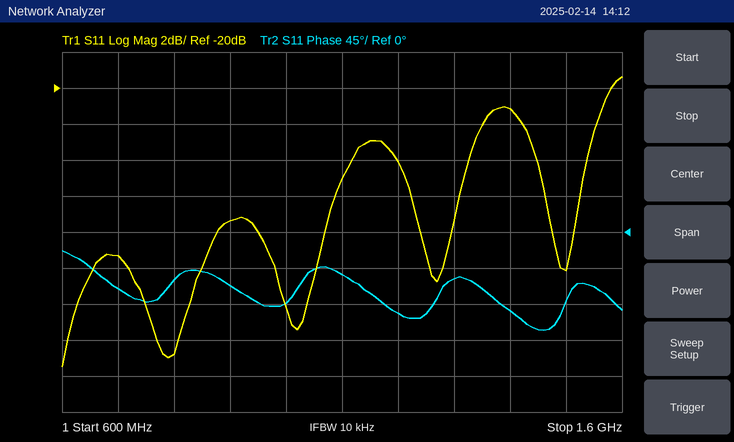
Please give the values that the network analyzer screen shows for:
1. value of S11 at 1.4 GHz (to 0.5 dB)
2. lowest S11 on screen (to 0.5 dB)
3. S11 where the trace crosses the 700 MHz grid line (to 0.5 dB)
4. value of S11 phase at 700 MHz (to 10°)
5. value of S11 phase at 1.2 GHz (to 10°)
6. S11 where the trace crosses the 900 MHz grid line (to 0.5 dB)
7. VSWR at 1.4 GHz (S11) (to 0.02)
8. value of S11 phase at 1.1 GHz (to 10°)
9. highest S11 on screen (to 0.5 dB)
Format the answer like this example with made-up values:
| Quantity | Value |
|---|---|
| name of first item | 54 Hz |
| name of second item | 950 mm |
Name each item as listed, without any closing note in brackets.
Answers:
| Quantity | Value |
|---|---|
| value of S11 at 1.4 GHz | -21.0 dB |
| lowest S11 on screen | -35.5 dB |
| S11 where the trace crosses the 700 MHz grid line | -29.5 dB |
| value of S11 phase at 700 MHz | -70° |
| value of S11 phase at 1.2 GHz | -100° |
| S11 where the trace crosses the 900 MHz grid line | -27.5 dB |
| VSWR at 1.4 GHz (S11) | 1.20 |
| value of S11 phase at 1.1 GHz | -50° |
| highest S11 on screen | -19.5 dB |
